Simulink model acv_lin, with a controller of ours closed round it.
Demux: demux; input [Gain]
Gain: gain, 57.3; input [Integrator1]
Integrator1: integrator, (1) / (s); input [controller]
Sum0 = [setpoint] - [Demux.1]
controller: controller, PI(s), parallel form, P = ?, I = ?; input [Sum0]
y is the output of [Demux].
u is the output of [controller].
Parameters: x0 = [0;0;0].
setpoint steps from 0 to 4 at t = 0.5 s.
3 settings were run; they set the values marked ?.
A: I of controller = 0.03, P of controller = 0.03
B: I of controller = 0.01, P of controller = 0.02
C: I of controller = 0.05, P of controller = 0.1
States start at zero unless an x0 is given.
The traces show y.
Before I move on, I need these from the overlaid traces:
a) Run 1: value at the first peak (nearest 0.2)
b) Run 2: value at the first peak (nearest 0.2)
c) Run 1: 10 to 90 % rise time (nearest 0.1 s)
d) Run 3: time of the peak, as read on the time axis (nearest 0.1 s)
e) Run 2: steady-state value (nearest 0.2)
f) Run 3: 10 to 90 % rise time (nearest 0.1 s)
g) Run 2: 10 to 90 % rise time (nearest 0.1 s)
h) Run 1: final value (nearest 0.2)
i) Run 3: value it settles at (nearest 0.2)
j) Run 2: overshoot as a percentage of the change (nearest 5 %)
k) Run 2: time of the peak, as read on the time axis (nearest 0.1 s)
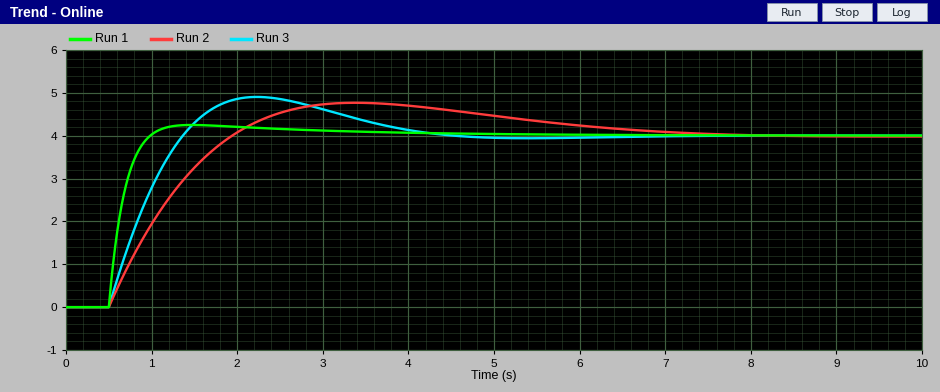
4.2
4.8
0.3 s
2.2 s
4.0
0.7 s
1.1 s
4.0
4.0
20 %
3.4 s
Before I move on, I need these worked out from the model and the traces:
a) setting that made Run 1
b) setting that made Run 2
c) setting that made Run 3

C
B
A
